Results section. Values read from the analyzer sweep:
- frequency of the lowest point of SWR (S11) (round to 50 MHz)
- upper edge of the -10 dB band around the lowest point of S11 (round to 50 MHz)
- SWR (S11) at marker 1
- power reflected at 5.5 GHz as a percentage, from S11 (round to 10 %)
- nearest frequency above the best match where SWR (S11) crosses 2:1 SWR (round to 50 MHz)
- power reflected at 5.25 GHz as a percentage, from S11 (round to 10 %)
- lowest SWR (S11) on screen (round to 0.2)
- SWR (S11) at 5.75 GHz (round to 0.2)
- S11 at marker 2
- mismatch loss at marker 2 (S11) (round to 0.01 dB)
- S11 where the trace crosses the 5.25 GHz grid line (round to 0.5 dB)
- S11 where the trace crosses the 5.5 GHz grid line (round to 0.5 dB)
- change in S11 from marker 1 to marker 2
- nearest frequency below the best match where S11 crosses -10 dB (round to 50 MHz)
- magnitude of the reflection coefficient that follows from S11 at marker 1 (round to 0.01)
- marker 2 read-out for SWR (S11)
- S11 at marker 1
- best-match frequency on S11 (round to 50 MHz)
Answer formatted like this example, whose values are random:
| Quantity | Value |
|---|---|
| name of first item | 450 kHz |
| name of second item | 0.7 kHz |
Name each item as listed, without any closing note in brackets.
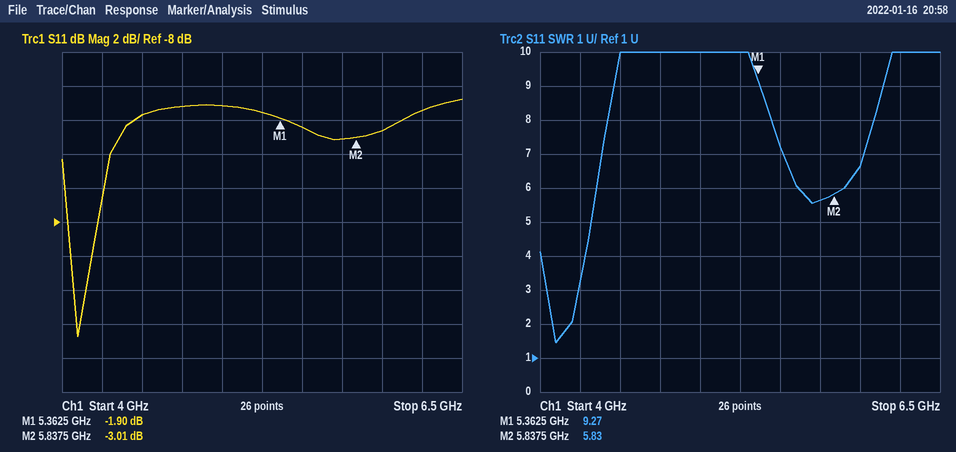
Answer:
| Quantity | Value |
|---|---|
| frequency of the lowest point of SWR (S11) | 4.10 GHz |
| upper edge of the -10 dB band around the lowest point of S11 | 4.20 GHz |
| SWR (S11) at marker 1 | 9.27 |
| power reflected at 5.5 GHz as a percentage, from S11 | 60 % |
| nearest frequency above the best match where SWR (S11) crosses 2:1 SWR | 4.20 GHz |
| power reflected at 5.25 GHz as a percentage, from S11 | 70 % |
| lowest SWR (S11) on screen | 1.4 |
| SWR (S11) at 5.75 GHz | 5.6 |
| S11 at marker 2 | -3.01 dB |
| mismatch loss at marker 2 (S11) | 3.01 dB |
| S11 where the trace crosses the 5.25 GHz grid line | -1.5 dB |
| S11 where the trace crosses the 5.5 GHz grid line | -2.5 dB |
| change in S11 from marker 1 to marker 2 | -1.11 dB |
| nearest frequency below the best match where S11 crosses -10 dB | 4.05 GHz |
| magnitude of the reflection coefficient that follows from S11 at marker 1 | 0.80 |
| marker 2 read-out for SWR | 5.83 |
| S11 at marker 1 | -1.90 dB |
| best-match frequency on S11 | 4.10 GHz |
